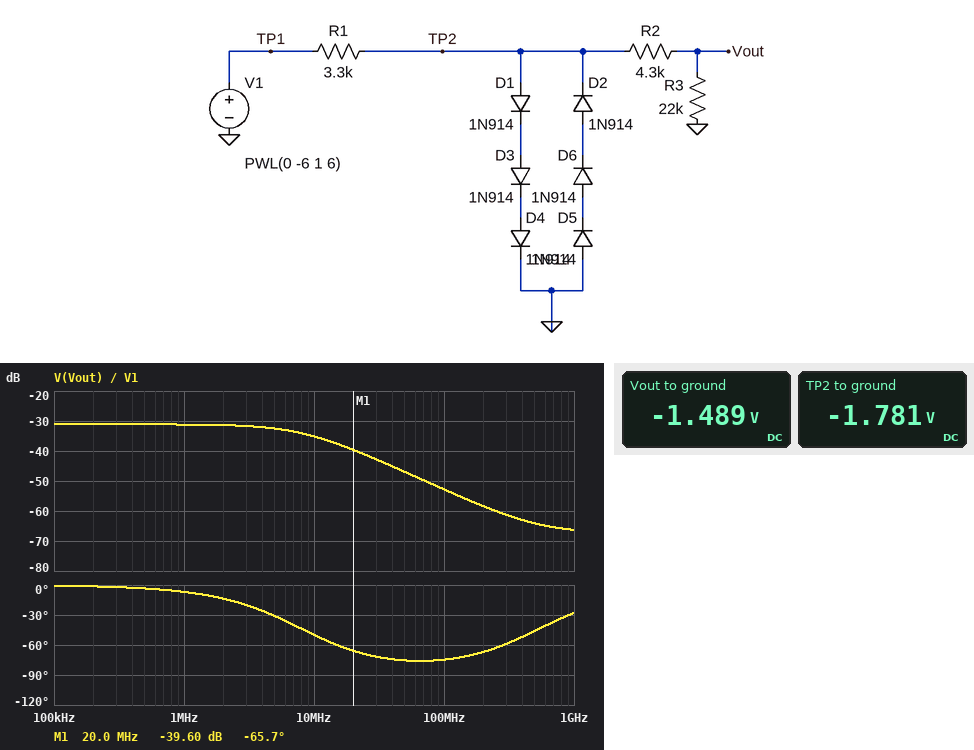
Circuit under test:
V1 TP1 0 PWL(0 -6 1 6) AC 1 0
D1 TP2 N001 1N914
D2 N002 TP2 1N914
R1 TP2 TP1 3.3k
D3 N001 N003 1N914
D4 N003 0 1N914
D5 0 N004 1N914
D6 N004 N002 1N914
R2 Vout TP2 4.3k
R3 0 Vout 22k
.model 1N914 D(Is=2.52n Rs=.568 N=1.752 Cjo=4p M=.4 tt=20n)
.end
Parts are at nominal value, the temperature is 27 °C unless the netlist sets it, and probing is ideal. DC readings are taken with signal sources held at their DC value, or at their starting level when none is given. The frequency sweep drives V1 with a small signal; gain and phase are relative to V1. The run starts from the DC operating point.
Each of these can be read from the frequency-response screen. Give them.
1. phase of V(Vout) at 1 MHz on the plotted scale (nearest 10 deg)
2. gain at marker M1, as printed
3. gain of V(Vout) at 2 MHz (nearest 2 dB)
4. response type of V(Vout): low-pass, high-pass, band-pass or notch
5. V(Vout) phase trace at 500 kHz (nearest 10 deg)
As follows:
-10 deg
-39.60 dB
-32 dB
low-pass
0 deg
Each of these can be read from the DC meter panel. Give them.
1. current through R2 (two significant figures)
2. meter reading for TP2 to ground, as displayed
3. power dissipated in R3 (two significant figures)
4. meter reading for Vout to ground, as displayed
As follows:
68 µA
-1.781 V
100 µW
-1.489 V
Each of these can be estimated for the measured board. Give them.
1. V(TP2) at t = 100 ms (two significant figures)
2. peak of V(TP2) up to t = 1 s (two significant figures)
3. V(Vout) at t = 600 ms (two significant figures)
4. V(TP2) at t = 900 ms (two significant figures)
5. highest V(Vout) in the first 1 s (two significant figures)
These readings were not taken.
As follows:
-1.7 V
1.8 V
880 mV
1.7 V
1.5 V
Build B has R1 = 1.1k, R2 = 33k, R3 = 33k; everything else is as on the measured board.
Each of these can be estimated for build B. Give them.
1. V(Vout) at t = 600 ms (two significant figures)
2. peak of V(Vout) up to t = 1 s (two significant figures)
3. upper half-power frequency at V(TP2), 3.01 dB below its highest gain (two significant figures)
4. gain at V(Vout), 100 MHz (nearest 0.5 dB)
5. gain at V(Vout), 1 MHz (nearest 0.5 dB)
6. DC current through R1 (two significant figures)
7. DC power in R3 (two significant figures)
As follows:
580 mV
970 mV
8.2 MHz
-56.0 dB
-35.5 dB
3.7 mA
28 µW
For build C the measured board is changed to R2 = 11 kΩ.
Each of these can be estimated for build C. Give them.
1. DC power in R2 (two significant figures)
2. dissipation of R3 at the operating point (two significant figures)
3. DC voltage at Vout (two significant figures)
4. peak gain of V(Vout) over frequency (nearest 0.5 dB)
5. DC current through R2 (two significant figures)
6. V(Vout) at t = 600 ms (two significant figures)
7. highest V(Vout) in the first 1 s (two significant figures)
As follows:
32 µW
64 µW
-1.2 V
-33.0 dB
54 µA
710 mV
1.2 V
